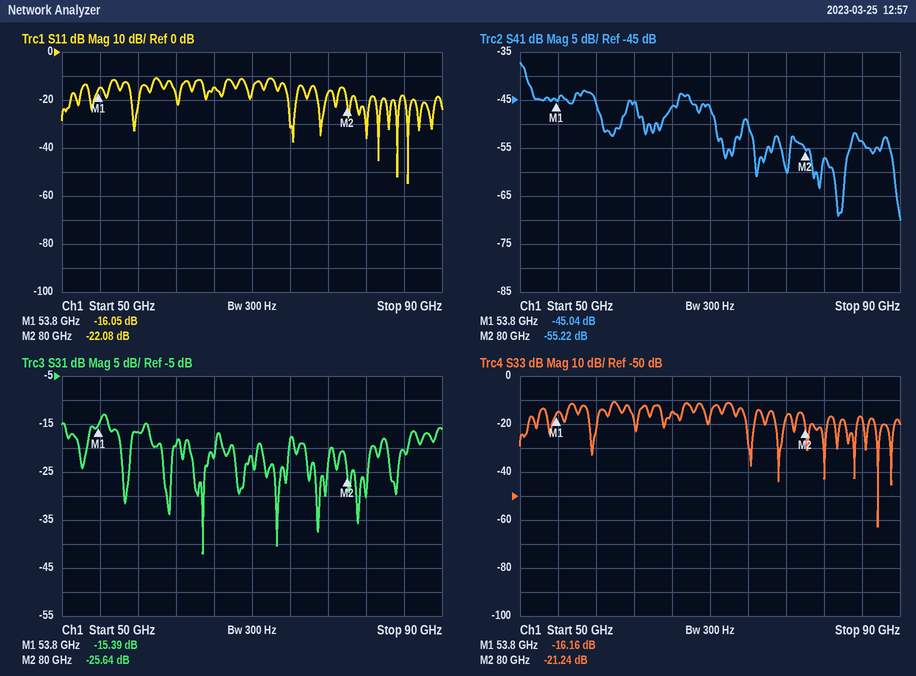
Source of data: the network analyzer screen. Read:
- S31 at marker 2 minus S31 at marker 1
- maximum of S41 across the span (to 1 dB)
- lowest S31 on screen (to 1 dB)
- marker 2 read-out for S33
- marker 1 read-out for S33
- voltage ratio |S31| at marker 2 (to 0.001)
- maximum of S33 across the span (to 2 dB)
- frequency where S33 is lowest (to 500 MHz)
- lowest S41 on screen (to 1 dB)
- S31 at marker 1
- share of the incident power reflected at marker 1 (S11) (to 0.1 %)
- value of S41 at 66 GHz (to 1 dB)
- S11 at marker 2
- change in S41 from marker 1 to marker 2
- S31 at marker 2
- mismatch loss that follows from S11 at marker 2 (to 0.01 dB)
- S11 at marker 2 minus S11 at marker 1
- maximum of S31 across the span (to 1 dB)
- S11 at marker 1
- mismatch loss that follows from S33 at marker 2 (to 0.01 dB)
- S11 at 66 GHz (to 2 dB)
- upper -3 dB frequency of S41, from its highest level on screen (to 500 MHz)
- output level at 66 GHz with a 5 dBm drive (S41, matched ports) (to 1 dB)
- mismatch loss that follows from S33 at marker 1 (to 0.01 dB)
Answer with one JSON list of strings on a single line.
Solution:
["-10.25 dB", "-37 dB", "-42 dB", "-21.24 dB", "-16.16 dB", "0.052", "-10 dB", "87.5 GHz", "-70 dB", "-15.39 dB", "2.5 %", "-46 dB", "-22.08 dB", "-10.18 dB", "-25.64 dB", "0.03 dB", "-6.03 dB", "-13 dB", "-16.05 dB", "0.03 dB", "-14 dB", "50.5 GHz", "-41 dBm", "0.11 dB"]
